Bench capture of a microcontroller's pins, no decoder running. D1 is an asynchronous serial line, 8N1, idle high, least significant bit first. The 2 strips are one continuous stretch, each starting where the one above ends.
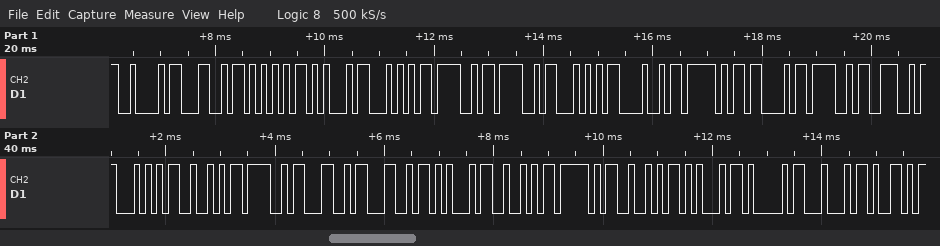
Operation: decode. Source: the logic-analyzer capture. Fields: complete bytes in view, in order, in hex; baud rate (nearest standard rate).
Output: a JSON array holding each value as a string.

["42 4C 55 45 54 4F 4F 54 48 5F 43 4F 4E 54 52 4F 4C 4C 45 52 5F 52 45 41 44 59", "9600 baud"]
